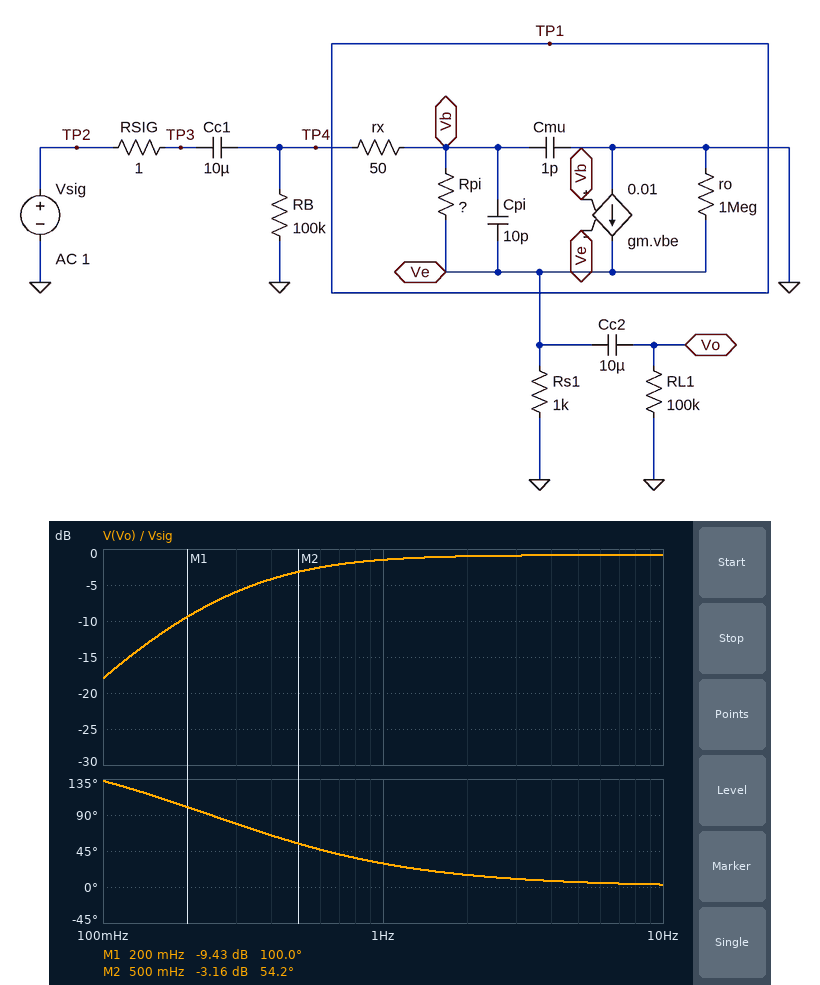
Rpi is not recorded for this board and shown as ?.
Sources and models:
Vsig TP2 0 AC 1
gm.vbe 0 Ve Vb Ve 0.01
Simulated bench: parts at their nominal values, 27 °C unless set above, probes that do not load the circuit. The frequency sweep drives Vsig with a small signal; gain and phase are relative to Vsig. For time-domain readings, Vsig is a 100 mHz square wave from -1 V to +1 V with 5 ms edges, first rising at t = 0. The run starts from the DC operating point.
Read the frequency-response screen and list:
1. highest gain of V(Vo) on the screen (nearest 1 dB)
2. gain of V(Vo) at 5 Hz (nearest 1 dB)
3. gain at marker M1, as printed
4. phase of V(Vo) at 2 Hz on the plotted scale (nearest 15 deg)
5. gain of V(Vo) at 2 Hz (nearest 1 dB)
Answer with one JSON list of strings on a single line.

["-1 dB", "-1 dB", "-9.43 dB", "15 deg", "-1 dB"]
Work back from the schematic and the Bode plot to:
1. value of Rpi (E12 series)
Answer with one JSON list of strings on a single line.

["6.8 kΩ"]
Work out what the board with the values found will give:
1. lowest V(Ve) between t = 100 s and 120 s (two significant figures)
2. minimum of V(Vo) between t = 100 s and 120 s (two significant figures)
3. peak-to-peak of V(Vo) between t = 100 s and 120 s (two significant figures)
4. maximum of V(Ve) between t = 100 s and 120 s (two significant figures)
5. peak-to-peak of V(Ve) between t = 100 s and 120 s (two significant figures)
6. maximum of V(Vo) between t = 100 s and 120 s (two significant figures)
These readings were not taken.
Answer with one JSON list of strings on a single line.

["-1.8 V", "-1.8 V", "3.6 V", "1.8 V", "3.6 V", "1.8 V"]
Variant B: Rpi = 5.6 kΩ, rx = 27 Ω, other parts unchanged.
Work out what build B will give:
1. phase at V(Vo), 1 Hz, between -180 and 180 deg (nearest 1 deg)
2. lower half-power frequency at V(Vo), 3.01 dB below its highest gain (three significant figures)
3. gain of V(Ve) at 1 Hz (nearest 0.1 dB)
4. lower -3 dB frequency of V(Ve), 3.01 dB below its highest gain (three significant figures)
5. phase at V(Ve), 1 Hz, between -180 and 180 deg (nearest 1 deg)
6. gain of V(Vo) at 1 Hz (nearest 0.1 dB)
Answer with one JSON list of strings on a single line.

["32 deg", "468 mHz", "-1.5 dB", "416 mHz", "23 deg", "-1.6 dB"]
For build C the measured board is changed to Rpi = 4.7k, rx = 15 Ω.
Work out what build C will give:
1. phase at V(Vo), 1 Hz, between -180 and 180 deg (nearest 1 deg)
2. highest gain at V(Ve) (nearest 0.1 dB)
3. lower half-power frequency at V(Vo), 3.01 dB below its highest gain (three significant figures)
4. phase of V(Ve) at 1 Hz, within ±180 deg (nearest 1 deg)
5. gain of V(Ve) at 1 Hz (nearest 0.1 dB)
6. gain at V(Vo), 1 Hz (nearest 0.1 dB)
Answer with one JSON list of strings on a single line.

["34 deg", "-0.8 dB", "512 mHz", "25 deg", "-1.7 dB", "-1.8 dB"]
